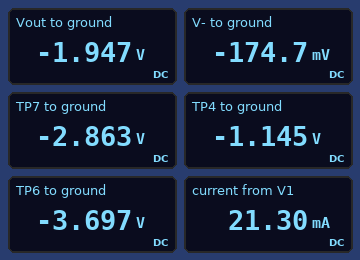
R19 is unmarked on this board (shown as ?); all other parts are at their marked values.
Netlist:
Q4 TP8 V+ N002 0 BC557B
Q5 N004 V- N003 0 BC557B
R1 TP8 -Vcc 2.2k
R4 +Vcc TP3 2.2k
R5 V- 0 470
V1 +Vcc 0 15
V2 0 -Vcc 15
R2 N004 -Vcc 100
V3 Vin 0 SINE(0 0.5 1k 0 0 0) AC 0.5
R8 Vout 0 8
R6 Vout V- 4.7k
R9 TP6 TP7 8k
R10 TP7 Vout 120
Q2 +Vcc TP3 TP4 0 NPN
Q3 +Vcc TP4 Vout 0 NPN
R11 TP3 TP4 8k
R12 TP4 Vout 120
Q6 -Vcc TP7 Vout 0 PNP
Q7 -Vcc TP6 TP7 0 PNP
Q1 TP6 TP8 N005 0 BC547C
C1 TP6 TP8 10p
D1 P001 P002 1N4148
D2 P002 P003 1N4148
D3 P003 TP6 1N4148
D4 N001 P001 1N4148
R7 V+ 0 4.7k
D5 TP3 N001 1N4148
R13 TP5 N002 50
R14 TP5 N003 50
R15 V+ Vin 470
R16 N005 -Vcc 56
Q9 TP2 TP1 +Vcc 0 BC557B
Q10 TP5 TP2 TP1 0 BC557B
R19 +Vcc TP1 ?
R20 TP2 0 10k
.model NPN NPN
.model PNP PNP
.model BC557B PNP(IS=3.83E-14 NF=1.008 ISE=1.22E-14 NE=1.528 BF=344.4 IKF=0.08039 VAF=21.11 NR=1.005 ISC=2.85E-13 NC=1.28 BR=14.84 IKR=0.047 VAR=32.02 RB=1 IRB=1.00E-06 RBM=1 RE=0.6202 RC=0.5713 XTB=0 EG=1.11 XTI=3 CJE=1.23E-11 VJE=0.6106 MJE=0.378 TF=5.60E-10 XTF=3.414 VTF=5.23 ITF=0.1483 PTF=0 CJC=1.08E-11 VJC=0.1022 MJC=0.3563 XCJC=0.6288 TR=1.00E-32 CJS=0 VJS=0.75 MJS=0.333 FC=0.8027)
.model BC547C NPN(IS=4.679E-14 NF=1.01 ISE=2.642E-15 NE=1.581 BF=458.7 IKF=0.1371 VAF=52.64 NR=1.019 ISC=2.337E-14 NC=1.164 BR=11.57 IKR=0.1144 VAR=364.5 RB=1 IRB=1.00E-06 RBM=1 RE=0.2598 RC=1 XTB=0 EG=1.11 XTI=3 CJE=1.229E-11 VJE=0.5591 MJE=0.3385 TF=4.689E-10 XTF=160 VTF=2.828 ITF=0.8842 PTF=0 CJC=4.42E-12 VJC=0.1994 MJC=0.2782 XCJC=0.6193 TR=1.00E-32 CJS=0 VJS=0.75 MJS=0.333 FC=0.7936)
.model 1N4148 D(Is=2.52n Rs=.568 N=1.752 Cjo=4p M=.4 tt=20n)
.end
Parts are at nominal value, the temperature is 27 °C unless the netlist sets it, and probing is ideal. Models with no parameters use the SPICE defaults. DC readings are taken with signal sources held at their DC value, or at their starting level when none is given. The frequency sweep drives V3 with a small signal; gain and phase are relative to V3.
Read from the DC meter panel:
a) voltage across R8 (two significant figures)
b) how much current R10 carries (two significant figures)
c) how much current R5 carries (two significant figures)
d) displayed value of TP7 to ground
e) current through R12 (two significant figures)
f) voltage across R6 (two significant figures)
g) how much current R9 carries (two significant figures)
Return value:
1.9 V
7.6 mA
370 µA
-2.863 V
6.7 mA
1.8 V
100 µA
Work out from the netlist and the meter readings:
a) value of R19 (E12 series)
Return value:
180 Ω
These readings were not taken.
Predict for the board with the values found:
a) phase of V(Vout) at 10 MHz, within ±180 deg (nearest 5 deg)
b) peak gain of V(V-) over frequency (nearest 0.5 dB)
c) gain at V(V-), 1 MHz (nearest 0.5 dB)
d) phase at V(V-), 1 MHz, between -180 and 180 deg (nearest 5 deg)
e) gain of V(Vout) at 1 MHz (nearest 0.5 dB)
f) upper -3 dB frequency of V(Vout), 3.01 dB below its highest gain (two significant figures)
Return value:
-95 deg
-1.0 dB
-1.0 dB
-10 deg
20.0 dB
11 MHz
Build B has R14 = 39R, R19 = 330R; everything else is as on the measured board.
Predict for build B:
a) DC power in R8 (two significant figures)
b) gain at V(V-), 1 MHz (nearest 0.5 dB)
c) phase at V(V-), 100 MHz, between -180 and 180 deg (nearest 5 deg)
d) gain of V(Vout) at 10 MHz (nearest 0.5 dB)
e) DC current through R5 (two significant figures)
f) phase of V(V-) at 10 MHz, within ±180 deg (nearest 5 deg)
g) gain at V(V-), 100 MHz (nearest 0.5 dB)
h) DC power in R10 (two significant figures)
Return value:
58 mW
-1.0 dB
-30 deg
17.0 dB
130 µA
-105 deg
-10.0 dB
6.6 mW
